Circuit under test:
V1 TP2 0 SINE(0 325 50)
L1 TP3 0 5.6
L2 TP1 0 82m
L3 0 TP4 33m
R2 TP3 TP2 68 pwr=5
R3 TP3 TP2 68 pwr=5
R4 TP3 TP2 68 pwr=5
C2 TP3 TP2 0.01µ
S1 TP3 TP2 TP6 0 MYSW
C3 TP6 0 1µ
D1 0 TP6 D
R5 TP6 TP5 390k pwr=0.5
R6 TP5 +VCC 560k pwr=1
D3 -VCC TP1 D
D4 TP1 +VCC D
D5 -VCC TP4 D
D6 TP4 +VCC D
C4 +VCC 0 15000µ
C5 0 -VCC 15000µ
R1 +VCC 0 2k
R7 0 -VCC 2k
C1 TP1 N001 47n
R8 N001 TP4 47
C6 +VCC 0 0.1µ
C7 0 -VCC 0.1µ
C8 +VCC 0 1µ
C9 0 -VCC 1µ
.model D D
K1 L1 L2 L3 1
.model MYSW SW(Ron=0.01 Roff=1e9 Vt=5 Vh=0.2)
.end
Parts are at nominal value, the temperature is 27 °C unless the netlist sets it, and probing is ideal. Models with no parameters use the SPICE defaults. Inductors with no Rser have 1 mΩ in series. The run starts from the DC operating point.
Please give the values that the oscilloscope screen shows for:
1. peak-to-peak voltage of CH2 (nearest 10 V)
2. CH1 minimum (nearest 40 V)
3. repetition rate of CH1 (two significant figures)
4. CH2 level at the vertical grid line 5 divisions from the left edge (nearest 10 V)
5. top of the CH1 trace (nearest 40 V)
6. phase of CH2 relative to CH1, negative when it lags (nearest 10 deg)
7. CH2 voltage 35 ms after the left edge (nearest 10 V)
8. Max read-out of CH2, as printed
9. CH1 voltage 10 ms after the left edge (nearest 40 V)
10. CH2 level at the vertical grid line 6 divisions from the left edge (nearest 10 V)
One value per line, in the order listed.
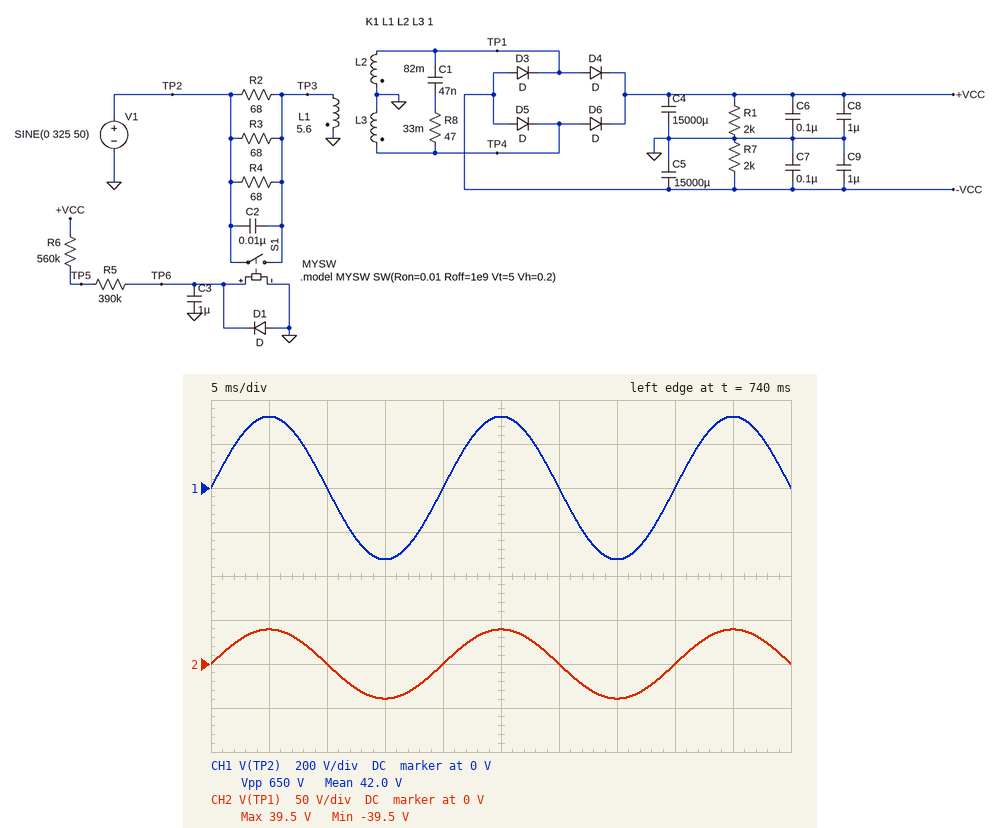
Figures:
80 V
-320 V
50 Hz
40 V
320 V
0 deg
-40 V
39.5 V
0 V
0 V
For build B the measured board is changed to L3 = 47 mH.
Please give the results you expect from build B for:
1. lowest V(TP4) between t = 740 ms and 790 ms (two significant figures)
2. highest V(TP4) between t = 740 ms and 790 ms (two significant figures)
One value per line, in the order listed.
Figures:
-30 V
30 V
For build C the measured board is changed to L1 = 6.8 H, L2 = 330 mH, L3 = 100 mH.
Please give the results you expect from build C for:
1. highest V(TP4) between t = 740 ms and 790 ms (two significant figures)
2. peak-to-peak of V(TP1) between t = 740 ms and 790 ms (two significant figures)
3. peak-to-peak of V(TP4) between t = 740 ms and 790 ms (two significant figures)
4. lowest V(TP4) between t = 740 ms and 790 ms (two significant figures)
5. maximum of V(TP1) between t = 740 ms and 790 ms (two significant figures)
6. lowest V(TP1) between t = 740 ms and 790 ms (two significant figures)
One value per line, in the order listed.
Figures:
39 V
140 V
79 V
-39 V
72 V
-72 V
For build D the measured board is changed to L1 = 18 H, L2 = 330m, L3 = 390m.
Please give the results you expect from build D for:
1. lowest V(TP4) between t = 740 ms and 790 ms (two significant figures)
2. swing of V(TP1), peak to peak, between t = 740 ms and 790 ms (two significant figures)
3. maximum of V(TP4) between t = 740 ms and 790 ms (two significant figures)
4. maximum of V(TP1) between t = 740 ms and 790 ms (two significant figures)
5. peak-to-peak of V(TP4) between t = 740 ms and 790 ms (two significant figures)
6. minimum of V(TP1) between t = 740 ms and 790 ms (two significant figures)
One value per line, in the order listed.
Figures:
-48 V
88 V
48 V
44 V
96 V
-44 V
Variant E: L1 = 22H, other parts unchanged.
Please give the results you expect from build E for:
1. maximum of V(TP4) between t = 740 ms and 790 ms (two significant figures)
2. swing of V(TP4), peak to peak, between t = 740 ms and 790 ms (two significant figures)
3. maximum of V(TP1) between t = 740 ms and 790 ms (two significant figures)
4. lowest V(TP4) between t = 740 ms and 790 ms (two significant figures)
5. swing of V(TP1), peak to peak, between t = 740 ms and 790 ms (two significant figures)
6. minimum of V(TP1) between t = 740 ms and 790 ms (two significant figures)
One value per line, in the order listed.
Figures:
13 V
25 V
20 V
-13 V
40 V
-20 V
